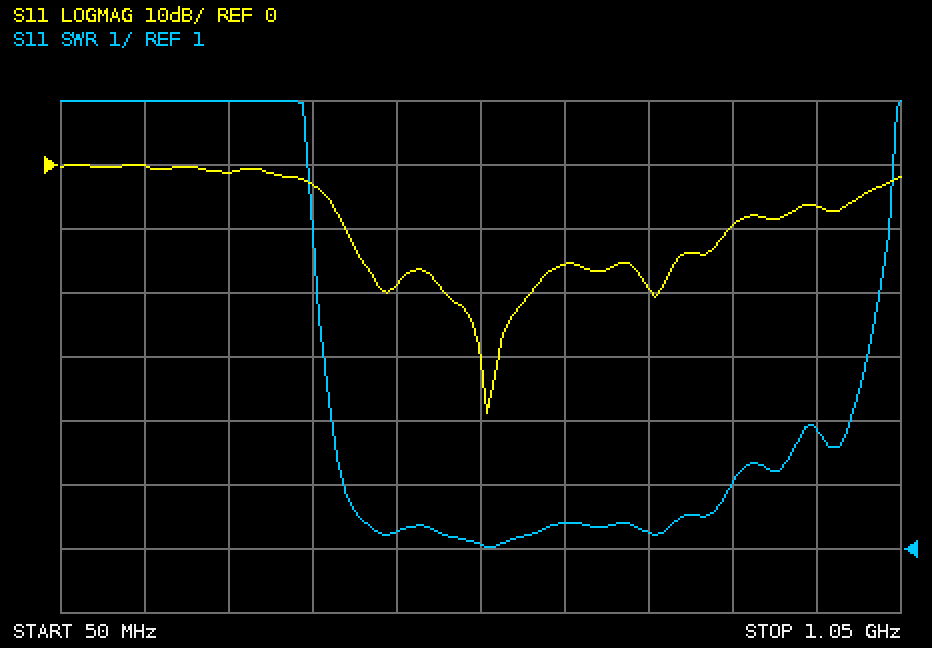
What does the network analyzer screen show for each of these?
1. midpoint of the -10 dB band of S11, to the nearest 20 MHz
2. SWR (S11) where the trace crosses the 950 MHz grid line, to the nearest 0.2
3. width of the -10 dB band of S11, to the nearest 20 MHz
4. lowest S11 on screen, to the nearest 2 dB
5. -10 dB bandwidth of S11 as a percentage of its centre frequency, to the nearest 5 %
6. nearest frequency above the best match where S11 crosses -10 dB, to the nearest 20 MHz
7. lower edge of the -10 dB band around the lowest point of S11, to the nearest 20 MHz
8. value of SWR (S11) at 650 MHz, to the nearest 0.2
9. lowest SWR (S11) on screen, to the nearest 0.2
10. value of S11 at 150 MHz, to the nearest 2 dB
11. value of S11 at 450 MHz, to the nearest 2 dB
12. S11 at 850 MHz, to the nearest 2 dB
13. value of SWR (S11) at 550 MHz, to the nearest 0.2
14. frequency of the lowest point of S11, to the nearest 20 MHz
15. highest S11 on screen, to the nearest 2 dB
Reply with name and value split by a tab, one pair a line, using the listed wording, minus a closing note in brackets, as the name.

midpoint of the -10 dB band of S11, to the nearest 20 MHz	620 MHz
SWR (S11) where the trace crosses the 950 MHz grid line, to the nearest 0.2	2.8
width of the -10 dB band of S11, to the nearest 20 MHz	460 MHz
lowest S11 on screen, to the nearest 2 dB	-38 dB
-10 dB bandwidth of S11 as a percentage of its centre frequency, to the nearest 5 %	75 %
nearest frequency above the best match where S11 crosses -10 dB, to the nearest 20 MHz	840 MHz
lower edge of the -10 dB band around the lowest point of S11, to the nearest 20 MHz	380 MHz
value of SWR (S11) at 650 MHz, to the nearest 0.2	1.4
lowest SWR (S11) on screen, to the nearest 0.2	1.0
value of S11 at 150 MHz, to the nearest 2 dB	0 dB
value of S11 at 450 MHz, to the nearest 2 dB	-18 dB
S11 at 850 MHz, to the nearest 2 dB	-10 dB
value of SWR (S11) at 550 MHz, to the nearest 0.2	1.0
frequency of the lowest point of S11, to the nearest 20 MHz	560 MHz
highest S11 on screen, to the nearest 2 dB	0 dB
